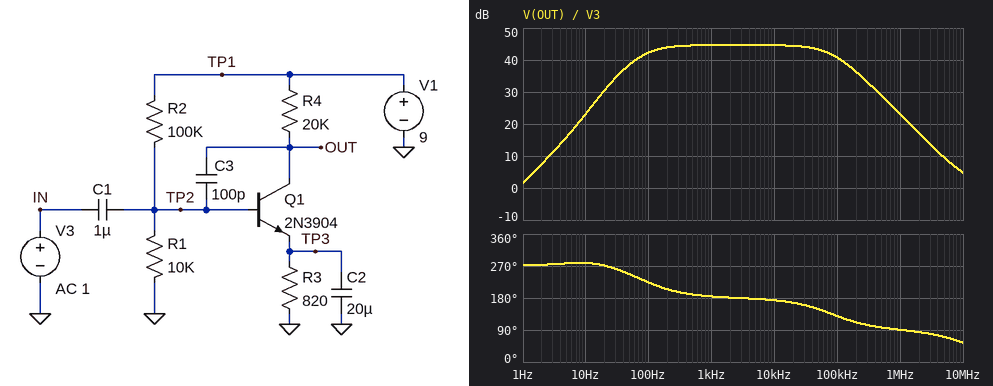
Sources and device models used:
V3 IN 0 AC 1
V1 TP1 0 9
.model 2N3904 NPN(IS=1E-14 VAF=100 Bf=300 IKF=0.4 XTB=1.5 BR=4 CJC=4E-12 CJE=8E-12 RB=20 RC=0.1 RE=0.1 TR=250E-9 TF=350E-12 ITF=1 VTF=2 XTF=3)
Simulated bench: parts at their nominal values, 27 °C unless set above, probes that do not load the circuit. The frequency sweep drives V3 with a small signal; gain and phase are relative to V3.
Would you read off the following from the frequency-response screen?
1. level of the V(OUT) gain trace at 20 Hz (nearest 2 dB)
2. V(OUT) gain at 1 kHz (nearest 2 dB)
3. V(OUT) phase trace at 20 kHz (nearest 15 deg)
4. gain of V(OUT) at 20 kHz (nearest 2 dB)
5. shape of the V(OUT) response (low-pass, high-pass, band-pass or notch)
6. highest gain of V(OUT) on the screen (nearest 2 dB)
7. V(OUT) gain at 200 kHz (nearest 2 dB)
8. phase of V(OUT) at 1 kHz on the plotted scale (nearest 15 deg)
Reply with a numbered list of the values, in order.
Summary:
1. 30 dB
2. 44 dB
3. 165 deg
4. 44 dB
5. band-pass
6. 44 dB
7. 36 dB
8. 180 deg
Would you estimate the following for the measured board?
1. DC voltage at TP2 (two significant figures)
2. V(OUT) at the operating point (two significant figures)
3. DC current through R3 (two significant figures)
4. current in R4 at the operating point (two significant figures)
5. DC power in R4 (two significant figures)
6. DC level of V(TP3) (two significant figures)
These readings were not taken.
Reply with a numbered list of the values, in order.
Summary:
1. 810 mV
2. 4.3 V
3. 240 µA
4. 240 µA
5. 1.1 mW
6. 190 mV
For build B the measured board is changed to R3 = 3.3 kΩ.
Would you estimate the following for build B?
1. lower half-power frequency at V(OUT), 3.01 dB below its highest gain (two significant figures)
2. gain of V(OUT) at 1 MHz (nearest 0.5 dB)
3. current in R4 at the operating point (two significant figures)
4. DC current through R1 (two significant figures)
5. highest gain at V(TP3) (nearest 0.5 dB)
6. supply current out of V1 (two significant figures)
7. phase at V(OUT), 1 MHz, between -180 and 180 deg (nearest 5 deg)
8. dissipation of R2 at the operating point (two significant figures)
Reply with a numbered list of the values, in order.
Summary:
1. 33 Hz
2. 12.5 dB
3. 70 µA
4. 82 µA
5. -6.0 dB
6. 150 µA
7. 80 deg
8. 670 µW
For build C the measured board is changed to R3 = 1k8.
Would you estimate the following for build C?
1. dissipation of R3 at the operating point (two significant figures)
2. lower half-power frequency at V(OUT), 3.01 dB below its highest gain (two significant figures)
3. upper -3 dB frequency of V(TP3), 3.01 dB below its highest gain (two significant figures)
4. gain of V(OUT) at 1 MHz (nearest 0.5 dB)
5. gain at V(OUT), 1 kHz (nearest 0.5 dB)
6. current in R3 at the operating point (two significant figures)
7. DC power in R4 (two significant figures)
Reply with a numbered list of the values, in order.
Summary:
1. 26 µW
2. 48 Hz
3. 70 Hz
4. 17.0 dB
5. 39.0 dB
6. 120 µA
7. 290 µW
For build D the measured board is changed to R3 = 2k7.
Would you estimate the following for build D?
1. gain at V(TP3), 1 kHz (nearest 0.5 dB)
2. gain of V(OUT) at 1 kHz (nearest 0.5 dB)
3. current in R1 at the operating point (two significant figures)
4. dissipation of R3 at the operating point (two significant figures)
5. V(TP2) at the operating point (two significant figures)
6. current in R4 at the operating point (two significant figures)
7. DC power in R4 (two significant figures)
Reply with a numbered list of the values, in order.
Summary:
1. -32.0 dB
2. 36.0 dB
3. 82 µA
4. 19 µW
5. 820 mV
6. 84 µA
7. 140 µW
